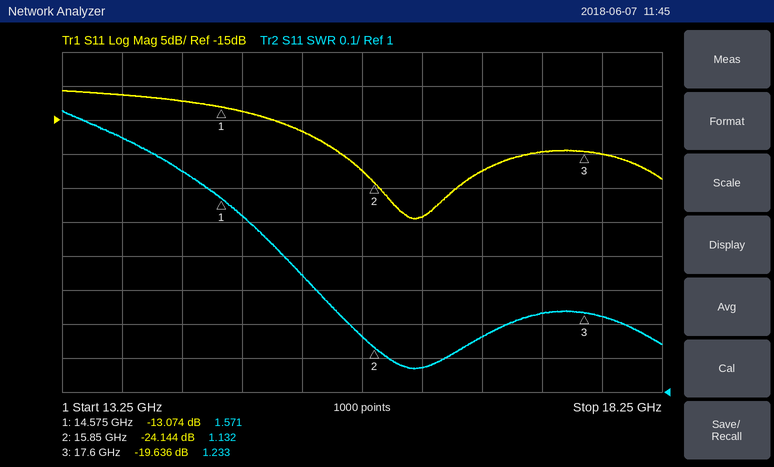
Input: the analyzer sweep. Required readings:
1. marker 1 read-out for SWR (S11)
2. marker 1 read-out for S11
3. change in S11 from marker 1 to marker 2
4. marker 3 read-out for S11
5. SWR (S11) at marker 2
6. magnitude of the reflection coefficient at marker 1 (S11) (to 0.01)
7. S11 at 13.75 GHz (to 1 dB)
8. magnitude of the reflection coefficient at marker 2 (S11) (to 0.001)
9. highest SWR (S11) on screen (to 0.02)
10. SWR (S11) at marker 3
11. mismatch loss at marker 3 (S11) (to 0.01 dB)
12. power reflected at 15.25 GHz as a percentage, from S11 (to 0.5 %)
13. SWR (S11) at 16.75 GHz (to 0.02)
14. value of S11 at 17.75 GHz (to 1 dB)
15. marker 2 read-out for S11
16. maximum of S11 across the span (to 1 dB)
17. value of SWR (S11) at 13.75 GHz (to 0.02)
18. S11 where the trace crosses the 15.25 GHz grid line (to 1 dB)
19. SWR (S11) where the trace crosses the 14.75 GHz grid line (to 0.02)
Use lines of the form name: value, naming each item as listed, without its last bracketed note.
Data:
marker 1 read-out for SWR: 1.571
marker 1 read-out for S11: -13.074 dB
change in S11 from marker 1 to marker 2: -11.070 dB
marker 3 read-out for S11: -19.636 dB
SWR (S11) at marker 2: 1.132
magnitude of the reflection coefficient at marker 1 (S11): 0.22
S11 at 13.75 GHz: -11 dB
magnitude of the reflection coefficient at marker 2 (S11): 0.062
highest SWR (S11) on screen: 1.82
SWR (S11) at marker 3: 1.233
mismatch loss at marker 3 (S11): 0.05 dB
power reflected at 15.25 GHz as a percentage, from S11: 2.0 %
SWR (S11) at 16.75 GHz: 1.16
value of S11 at 17.75 GHz: -20 dB
marker 2 read-out for S11: -24.144 dB
maximum of S11 across the span: -11 dB
value of SWR (S11) at 13.75 GHz: 1.74
S11 where the trace crosses the 15.25 GHz grid line: -17 dB
SWR (S11) where the trace crosses the 14.75 GHz grid line: 1.52
